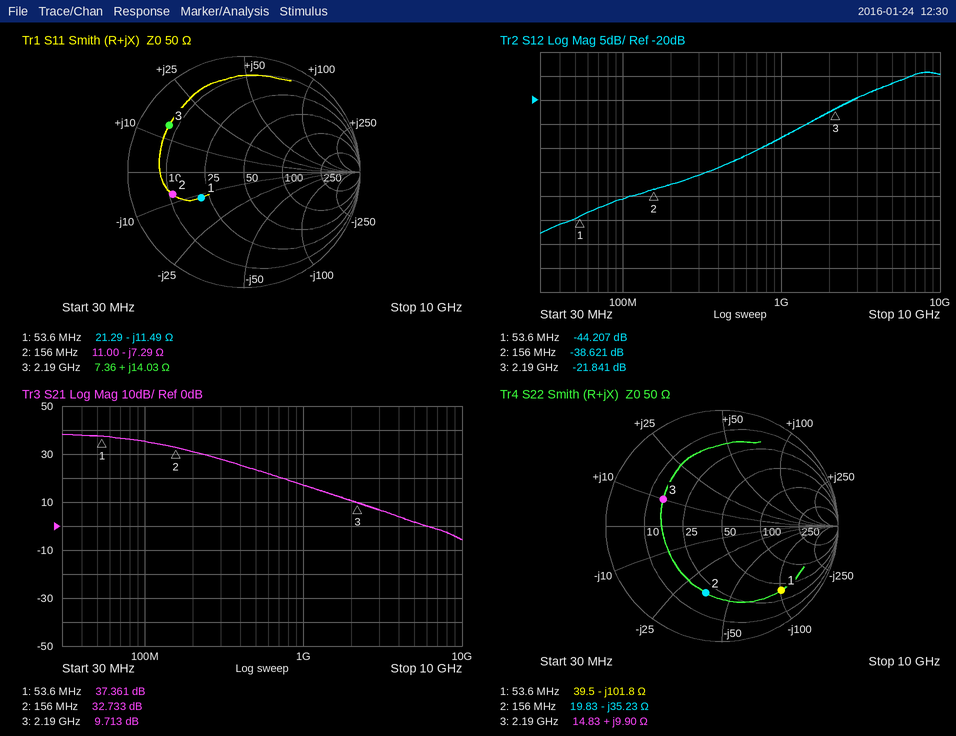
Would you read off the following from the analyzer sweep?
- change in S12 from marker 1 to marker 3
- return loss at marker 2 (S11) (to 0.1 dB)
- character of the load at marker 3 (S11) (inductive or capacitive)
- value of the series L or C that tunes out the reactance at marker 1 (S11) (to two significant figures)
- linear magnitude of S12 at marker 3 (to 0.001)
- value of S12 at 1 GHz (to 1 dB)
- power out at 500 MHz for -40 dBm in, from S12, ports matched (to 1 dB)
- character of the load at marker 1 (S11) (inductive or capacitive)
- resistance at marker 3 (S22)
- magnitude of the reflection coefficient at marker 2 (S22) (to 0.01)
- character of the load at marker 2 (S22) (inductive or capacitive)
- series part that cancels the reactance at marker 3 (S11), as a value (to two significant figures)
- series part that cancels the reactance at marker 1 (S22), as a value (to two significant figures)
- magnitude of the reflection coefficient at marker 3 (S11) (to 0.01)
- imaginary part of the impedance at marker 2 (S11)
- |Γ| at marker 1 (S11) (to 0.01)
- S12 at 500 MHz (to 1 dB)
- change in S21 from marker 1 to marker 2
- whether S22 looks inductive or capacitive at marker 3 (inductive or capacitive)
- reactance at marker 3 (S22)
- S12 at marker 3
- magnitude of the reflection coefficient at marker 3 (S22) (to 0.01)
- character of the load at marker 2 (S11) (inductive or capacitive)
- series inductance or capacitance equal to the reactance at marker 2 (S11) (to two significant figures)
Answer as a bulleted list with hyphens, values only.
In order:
- 22.366 dB
- 3.8 dB
- inductive
- 34 nH
- 0.081
- -28 dB
- -73 dBm
- capacitive
- 14.83 Ω
- 0.59
- capacitive
- 5.2 pF
- 300 nH
- 0.76
- -7.29 Ω
- 0.43
- -33 dB
- -4.628 dB
- inductive
- +9.90 Ω
- -21.841 dB
- 0.56
- capacitive
- 140 pF
